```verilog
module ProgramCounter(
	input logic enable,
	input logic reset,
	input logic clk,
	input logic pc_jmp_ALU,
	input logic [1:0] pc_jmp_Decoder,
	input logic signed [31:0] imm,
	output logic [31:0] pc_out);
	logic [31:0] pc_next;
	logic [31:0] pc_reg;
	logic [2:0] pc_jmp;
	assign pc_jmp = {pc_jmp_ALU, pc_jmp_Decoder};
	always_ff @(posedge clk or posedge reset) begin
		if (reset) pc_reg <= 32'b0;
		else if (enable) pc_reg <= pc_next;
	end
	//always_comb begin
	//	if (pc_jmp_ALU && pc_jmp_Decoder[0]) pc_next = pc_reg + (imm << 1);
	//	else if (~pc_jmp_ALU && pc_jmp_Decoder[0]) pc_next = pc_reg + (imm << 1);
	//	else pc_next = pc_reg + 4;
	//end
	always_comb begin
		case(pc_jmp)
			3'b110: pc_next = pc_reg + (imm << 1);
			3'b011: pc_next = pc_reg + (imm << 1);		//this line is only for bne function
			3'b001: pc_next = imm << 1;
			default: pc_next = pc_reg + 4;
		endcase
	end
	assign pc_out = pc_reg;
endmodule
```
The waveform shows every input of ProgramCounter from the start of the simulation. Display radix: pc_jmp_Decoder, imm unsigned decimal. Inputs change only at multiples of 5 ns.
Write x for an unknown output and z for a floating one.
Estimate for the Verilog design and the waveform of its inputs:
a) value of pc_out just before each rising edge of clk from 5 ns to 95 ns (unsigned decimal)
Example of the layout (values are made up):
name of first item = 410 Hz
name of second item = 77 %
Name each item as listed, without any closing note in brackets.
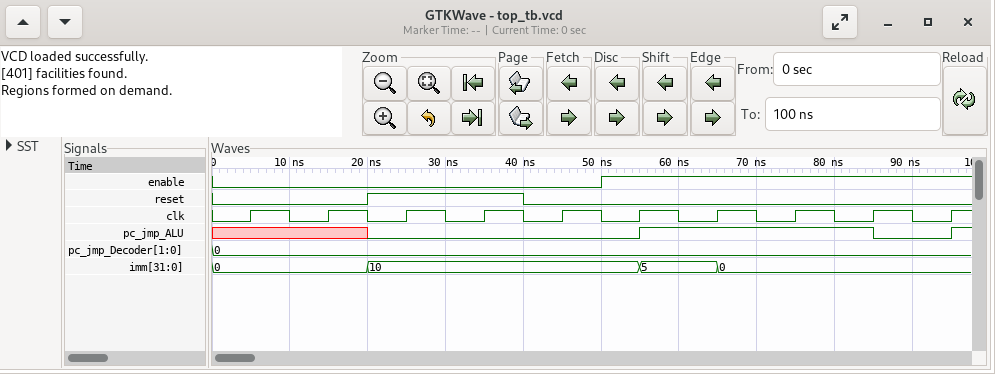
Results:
value of pc_out just before each rising edge of clk from 5 ns to 95 ns = x, x, 0, 0, 0, 0, 4, 8, 12, 16
